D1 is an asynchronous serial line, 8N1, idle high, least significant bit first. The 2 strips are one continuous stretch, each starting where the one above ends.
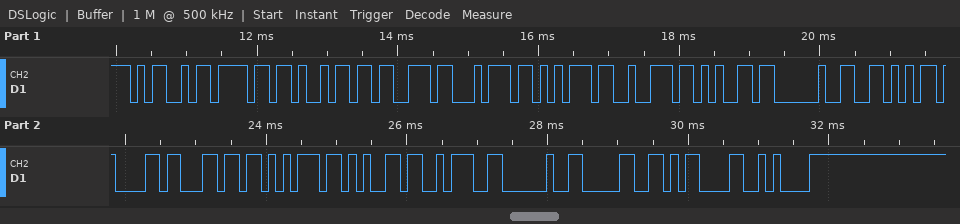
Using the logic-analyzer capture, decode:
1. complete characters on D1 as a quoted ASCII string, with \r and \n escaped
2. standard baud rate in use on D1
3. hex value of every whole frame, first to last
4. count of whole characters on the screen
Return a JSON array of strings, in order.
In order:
["\"Moisture Value: 0\\r\\n\"", "9600 baud", "4D 6F 69 73 74 75 72 65 20 56 61 6C 75 65 3A 20 30 0D 0A", "19"]
